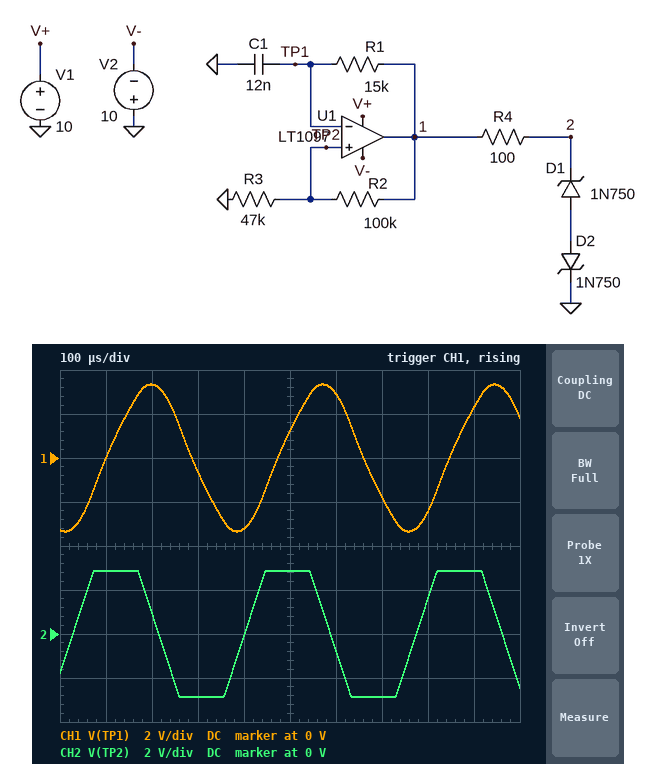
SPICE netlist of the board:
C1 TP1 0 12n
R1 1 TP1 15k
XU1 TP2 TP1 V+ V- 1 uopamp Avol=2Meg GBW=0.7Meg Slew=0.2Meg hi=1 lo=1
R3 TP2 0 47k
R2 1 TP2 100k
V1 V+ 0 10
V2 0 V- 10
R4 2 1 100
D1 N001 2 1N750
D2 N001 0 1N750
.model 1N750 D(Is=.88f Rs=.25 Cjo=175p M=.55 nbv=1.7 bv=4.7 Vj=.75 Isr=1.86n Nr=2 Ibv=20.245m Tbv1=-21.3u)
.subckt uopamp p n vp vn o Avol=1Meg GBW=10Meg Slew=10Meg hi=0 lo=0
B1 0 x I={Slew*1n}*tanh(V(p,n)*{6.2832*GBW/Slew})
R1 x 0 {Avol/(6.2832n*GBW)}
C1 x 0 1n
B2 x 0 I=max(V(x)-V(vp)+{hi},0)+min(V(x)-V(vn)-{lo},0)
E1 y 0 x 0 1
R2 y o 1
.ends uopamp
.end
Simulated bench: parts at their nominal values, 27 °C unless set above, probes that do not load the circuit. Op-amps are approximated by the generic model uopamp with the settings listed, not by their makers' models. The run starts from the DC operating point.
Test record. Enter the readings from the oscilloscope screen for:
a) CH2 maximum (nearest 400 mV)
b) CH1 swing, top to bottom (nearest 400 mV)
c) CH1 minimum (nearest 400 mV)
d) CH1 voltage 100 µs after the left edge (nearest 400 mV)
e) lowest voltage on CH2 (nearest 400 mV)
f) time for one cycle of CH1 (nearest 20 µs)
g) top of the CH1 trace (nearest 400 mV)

2.8 V
6.8 V
-3.2 V
0 V
-2.8 V
380 µs
3.2 V
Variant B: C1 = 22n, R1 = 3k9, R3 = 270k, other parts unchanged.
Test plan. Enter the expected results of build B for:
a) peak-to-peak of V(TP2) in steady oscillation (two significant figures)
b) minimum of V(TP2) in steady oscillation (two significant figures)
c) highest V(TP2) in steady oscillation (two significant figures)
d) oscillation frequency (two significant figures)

13 V
-6.5 V
6.5 V
2.3 kHz
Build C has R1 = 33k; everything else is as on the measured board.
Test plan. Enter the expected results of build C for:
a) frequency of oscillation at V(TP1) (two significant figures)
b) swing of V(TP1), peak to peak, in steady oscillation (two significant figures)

1.5 kHz
6.2 V
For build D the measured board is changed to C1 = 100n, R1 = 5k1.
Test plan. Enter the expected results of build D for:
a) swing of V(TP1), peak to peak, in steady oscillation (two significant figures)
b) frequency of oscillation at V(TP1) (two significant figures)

6.1 V
1.2 kHz
